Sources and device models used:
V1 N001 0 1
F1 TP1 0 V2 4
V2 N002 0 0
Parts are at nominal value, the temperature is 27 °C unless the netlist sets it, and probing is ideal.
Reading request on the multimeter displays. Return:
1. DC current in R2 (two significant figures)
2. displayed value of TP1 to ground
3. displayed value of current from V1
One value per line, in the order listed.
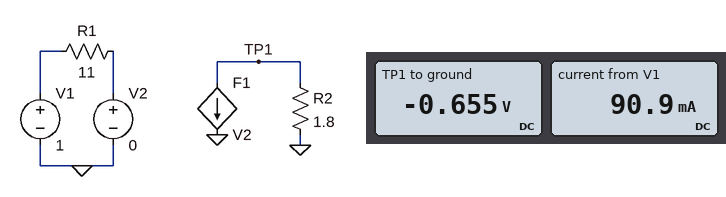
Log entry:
360 mA
-0.655 V
90.9 mA
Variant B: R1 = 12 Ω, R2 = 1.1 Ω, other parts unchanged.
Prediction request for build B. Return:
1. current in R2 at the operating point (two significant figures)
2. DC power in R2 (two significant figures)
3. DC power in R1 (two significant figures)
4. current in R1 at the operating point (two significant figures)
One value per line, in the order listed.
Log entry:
330 mA
120 mW
83 mW
83 mA
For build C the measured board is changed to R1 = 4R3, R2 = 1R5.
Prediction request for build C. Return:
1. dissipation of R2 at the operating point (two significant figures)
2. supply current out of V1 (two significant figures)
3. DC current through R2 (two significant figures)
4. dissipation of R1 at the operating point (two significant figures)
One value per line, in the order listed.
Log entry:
1.3 W
230 mA
930 mA
230 mW
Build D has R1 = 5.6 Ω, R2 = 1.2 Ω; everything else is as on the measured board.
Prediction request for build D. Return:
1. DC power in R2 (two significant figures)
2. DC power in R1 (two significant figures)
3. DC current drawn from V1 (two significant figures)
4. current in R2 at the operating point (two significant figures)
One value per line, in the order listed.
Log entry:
610 mW
180 mW
180 mA
710 mA
